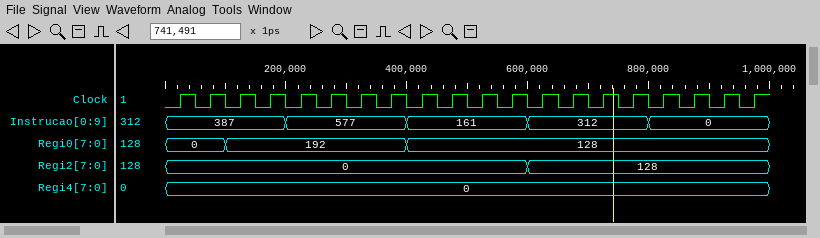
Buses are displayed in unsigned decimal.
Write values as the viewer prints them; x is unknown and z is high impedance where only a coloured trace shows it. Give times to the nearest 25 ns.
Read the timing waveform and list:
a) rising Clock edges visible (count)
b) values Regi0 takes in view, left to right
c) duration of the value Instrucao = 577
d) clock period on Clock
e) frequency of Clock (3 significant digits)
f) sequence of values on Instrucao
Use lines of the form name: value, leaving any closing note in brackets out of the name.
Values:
rising Clock edges visible: 20
values Regi0 takes in view, left to right: 0, 192, 128
duration of the value Instrucao = 577: 200 ns
clock period on Clock: 50 ns
frequency of Clock: 20.0 MHz
sequence of values on Instrucao: 387, 577, 161, 312, 0
